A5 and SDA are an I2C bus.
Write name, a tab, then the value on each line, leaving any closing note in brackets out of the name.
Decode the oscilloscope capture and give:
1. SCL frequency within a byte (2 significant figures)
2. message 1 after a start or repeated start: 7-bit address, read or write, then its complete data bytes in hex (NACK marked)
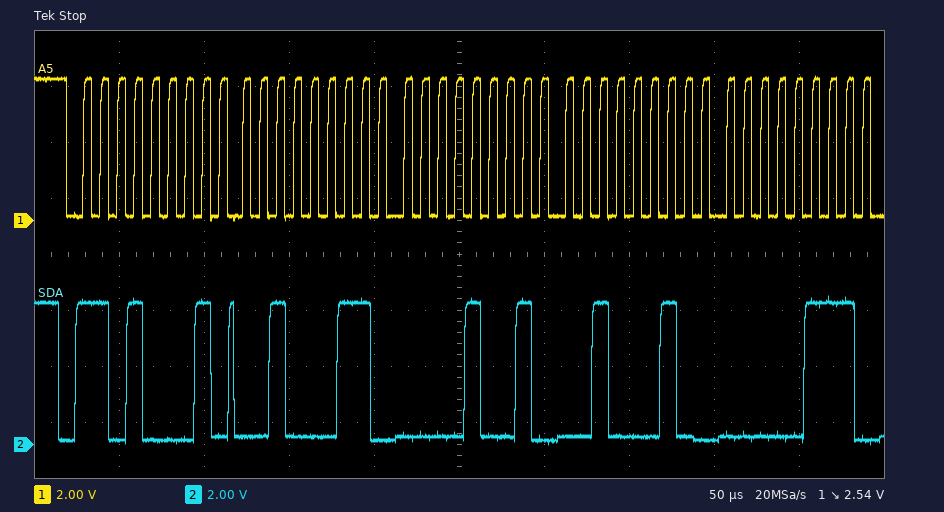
SCL frequency within a byte	100 kHz
message 1 after a start or repeated start: 7-bit address, read or write, then its complete data bytes in hex	0x68 read: 23 09 22 07
